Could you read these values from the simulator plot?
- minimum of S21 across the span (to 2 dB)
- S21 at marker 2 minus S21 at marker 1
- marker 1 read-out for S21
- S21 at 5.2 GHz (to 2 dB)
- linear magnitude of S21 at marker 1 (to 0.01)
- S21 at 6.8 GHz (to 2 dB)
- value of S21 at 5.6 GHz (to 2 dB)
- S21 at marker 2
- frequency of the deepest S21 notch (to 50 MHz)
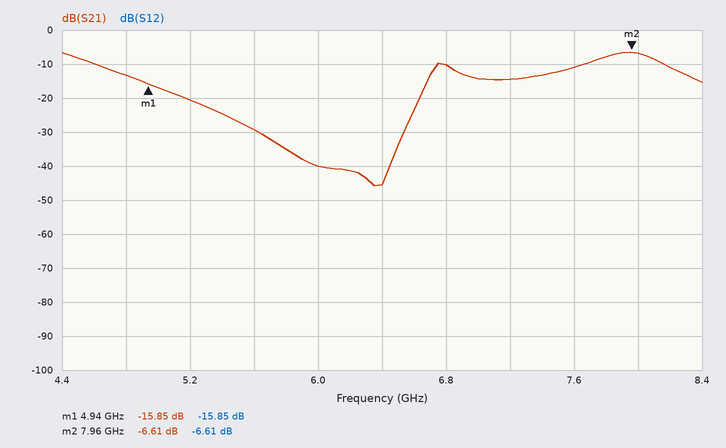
-46 dB
9.24 dB
-15.85 dB
-20 dB
0.16
-10 dB
-30 dB
-6.61 dB
6.35 GHz
